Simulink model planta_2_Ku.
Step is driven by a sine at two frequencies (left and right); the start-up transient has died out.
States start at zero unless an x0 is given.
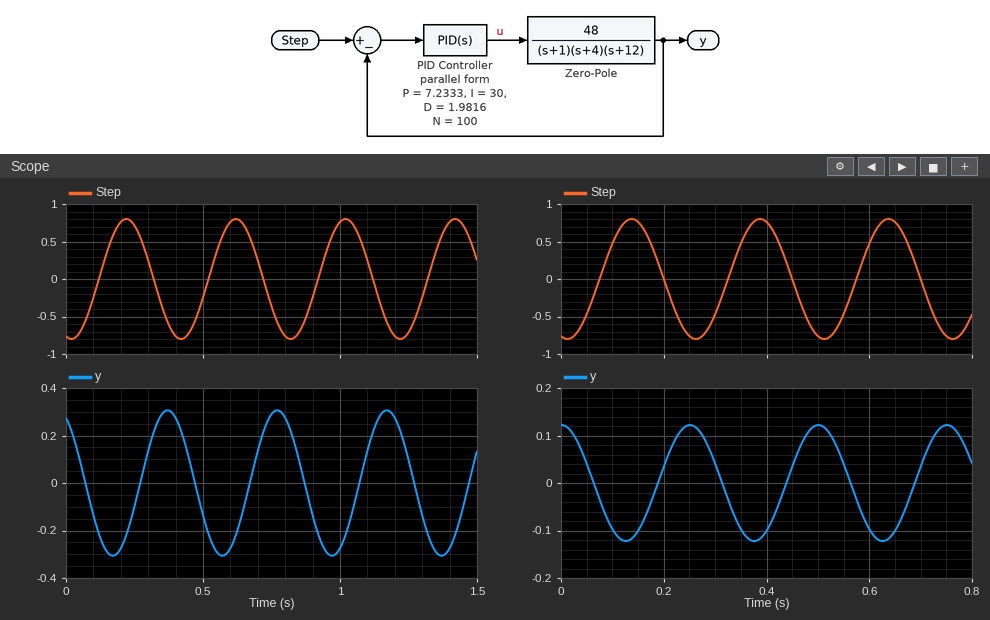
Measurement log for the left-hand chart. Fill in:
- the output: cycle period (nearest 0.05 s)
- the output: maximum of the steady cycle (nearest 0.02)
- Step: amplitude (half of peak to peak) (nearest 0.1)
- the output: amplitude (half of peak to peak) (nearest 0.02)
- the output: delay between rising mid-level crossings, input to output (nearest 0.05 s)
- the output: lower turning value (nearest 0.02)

0.40 s
0.30
0.8
0.30
0.15 s
-0.30
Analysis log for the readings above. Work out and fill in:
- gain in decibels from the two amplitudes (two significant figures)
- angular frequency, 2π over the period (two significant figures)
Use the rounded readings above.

-8.5 dB
16 rad/s
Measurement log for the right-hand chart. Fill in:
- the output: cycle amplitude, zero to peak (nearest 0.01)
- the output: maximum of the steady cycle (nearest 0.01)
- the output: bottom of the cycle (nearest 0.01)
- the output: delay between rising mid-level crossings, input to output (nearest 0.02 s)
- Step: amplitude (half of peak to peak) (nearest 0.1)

0.12
0.12
-0.12
0.12 s
0.8
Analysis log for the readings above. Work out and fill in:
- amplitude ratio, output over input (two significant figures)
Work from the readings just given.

0.15
